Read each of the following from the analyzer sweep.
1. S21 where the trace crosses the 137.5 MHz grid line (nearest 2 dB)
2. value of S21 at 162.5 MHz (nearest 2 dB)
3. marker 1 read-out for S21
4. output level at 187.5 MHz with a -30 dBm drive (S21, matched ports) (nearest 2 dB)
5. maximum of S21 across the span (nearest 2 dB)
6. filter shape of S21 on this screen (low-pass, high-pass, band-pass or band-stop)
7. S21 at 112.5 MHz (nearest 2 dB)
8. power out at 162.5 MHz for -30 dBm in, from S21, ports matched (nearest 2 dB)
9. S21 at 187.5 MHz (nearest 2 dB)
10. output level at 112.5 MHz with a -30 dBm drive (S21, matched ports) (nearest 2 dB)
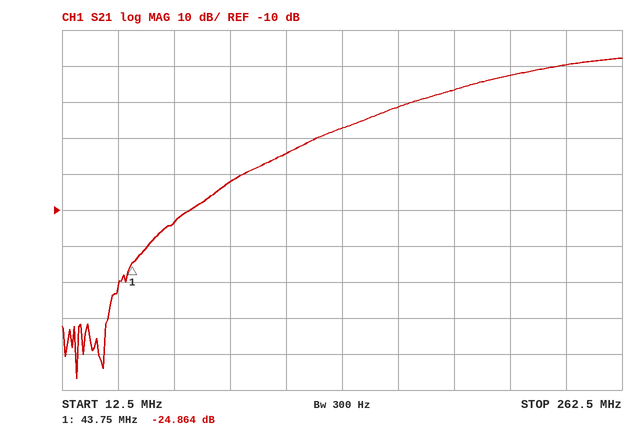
12 dB
18 dB
-24.864 dB
-6 dBm
32 dB
high-pass
6 dB
-12 dBm
24 dB
-24 dBm
